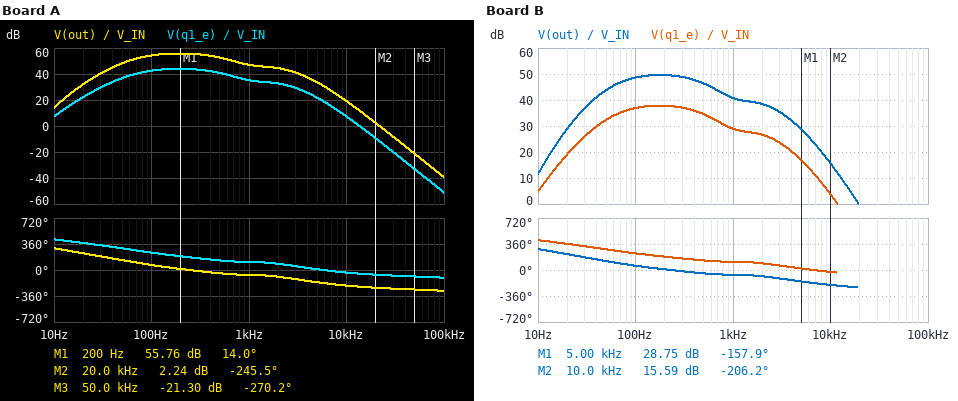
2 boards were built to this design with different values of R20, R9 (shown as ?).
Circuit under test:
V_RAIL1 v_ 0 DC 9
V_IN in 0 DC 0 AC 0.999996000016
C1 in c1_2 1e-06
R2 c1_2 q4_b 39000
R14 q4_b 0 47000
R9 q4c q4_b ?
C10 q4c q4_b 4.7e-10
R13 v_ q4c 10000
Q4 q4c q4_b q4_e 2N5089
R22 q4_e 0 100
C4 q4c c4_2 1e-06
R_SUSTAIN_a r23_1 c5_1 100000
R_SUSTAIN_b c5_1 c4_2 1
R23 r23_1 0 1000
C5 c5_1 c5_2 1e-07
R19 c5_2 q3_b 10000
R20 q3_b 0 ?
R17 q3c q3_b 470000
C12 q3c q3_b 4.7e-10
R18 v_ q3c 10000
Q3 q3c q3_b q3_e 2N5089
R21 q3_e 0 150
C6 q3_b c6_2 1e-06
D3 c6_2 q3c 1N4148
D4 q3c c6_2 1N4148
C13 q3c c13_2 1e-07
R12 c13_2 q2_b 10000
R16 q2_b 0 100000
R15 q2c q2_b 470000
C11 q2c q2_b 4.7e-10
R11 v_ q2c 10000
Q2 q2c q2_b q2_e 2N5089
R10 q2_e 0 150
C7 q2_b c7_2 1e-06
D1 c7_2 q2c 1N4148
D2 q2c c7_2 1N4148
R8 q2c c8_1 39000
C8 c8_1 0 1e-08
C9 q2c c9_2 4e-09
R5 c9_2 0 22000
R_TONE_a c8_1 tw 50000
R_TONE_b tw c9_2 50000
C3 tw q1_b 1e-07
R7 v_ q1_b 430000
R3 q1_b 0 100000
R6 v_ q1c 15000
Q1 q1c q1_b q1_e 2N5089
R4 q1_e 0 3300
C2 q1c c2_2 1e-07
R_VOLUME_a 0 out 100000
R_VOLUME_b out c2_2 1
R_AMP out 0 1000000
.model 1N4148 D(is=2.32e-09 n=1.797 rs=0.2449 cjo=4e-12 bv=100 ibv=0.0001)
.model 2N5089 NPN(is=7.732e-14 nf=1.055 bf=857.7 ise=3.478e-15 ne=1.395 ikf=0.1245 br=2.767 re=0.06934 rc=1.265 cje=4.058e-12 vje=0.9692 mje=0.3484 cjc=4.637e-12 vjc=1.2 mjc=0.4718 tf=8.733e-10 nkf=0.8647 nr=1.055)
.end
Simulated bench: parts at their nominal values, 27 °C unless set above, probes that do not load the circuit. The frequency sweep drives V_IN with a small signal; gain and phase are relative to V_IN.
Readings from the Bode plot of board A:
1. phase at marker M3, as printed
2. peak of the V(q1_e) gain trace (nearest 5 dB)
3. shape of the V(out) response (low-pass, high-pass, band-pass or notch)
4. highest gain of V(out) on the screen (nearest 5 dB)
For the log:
-270.2 deg
45 dB
band-pass
55 dB
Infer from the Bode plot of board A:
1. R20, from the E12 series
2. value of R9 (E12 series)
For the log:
39 kΩ
180 kΩ
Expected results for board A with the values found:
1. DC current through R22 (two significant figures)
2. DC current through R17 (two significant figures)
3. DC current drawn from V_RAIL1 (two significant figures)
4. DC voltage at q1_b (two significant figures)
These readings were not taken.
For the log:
550 µA
15 µA
1.5 mA
1.7 V
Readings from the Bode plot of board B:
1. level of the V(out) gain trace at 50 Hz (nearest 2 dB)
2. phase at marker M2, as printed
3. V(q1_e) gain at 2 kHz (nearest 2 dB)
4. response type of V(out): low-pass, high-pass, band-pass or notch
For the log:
44 dB
-206.2 deg
26 dB
band-pass
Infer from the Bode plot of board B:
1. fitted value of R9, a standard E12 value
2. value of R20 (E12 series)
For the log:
680 kΩ
33 kΩ
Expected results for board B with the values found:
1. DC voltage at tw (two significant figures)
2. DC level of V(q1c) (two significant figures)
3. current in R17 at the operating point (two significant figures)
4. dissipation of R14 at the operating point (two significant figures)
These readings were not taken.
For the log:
1.9 V
4.2 V
17 µA
6.4 µW
